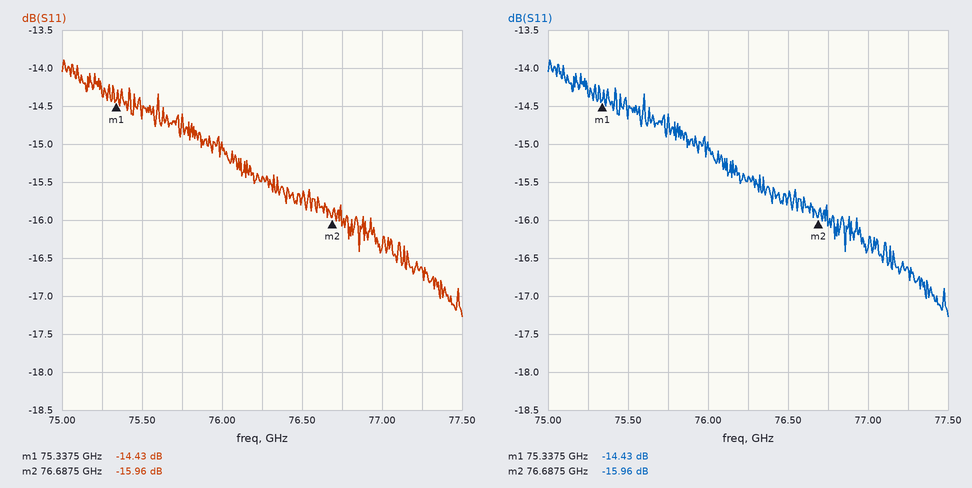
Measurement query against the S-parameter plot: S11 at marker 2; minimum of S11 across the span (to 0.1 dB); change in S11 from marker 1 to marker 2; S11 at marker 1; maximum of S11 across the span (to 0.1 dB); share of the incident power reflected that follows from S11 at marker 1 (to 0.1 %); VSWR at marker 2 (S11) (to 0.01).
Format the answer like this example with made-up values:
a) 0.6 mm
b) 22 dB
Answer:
a) -15.96 dB
b) -17.3 dB
c) -1.53 dB
d) -14.43 dB
e) -13.9 dB
f) 3.6 %
g) 1.38
